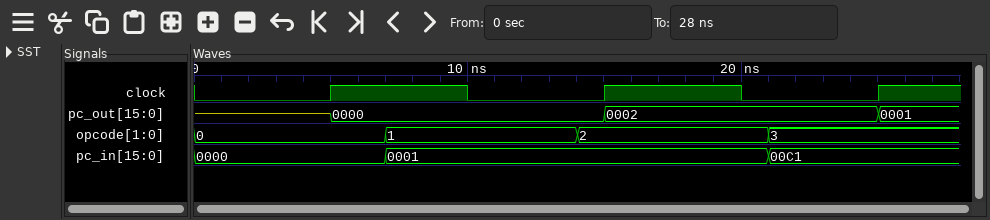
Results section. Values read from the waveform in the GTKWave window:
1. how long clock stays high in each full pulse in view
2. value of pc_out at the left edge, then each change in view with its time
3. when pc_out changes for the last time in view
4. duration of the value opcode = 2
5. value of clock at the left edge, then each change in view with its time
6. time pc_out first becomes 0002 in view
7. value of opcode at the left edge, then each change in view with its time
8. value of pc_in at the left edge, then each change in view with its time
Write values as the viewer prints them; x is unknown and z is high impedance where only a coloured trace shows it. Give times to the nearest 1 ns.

5 ns, 5 ns
z, 0000 at 5 ns, 0002 at 15 ns, 0001 at 25 ns
25 ns
7 ns
0, 1 at 5 ns, 0 at 10 ns, 1 at 15 ns, 0 at 20 ns, 1 at 25 ns
15 ns
0, 1 at 7 ns, 2 at 14 ns, 3 at 21 ns
0000, 0001 at 7 ns, 00C1 at 21 ns
